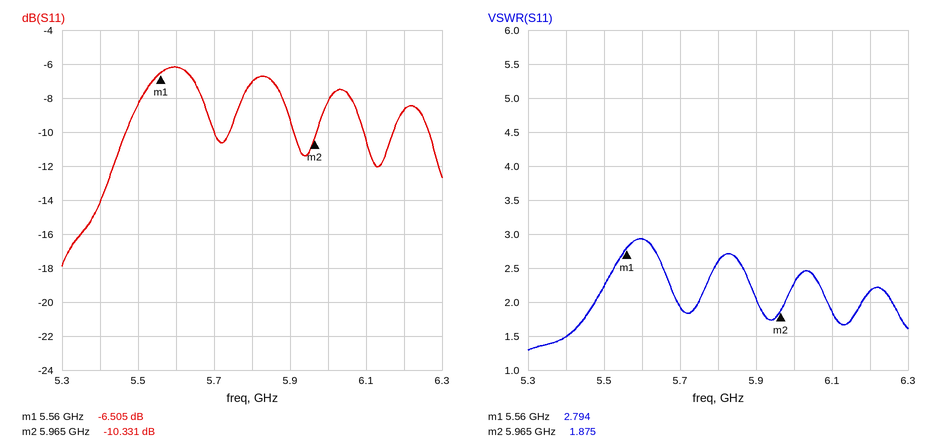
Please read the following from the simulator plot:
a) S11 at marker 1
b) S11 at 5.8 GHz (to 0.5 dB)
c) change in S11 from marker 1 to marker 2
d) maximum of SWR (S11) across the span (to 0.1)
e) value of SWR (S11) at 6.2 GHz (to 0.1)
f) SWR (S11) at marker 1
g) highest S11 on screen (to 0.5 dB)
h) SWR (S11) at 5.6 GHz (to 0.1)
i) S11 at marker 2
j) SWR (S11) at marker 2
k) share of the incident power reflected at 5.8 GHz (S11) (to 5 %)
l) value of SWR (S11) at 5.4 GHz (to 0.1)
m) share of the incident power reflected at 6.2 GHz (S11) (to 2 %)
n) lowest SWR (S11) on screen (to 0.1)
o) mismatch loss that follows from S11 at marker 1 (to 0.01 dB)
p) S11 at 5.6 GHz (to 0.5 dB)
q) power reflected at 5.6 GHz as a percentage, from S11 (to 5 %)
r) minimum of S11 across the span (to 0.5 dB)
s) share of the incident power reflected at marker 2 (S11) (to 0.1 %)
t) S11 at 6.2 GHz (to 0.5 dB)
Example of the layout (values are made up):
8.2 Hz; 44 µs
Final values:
-6.505 dB; -7.0 dB; -3.826 dB; 2.9; 2.2; 2.794; -6.0 dB; 2.9; -10.331 dB; 1.875; 20 %; 1.5; 14 %; 1.3; 1.10 dB; -6.0 dB; 25 %; -18.0 dB; 9.3 %; -8.5 dB
